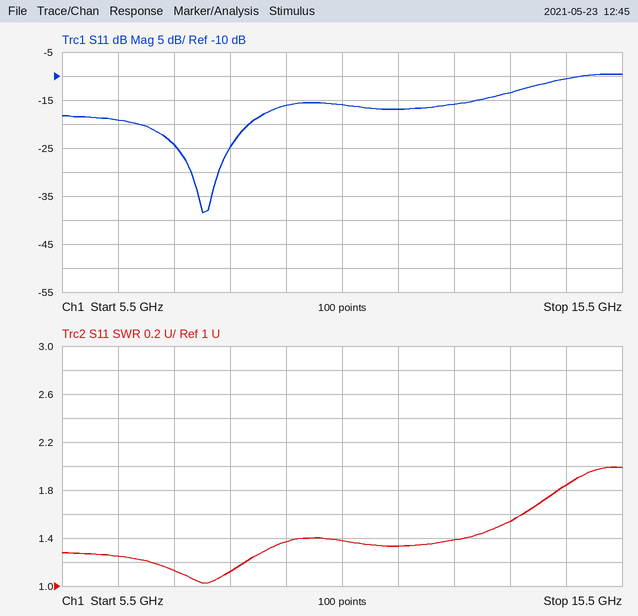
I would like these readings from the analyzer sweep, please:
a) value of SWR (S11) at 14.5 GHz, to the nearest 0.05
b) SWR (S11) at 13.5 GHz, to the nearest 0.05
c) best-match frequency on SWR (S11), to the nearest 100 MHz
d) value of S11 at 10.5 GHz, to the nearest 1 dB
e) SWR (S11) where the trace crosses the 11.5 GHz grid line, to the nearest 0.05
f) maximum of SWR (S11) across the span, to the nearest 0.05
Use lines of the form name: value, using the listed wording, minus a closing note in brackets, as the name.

value of SWR (S11) at 14.5 GHz, to the nearest 0.05: 1.85
SWR (S11) at 13.5 GHz, to the nearest 0.05: 1.55
best-match frequency on SWR (S11), to the nearest 100 MHz: 8.0 GHz
value of S11 at 10.5 GHz, to the nearest 1 dB: -16 dB
SWR (S11) where the trace crosses the 11.5 GHz grid line, to the nearest 0.05: 1.35
maximum of SWR (S11) across the span, to the nearest 0.05: 2.00
